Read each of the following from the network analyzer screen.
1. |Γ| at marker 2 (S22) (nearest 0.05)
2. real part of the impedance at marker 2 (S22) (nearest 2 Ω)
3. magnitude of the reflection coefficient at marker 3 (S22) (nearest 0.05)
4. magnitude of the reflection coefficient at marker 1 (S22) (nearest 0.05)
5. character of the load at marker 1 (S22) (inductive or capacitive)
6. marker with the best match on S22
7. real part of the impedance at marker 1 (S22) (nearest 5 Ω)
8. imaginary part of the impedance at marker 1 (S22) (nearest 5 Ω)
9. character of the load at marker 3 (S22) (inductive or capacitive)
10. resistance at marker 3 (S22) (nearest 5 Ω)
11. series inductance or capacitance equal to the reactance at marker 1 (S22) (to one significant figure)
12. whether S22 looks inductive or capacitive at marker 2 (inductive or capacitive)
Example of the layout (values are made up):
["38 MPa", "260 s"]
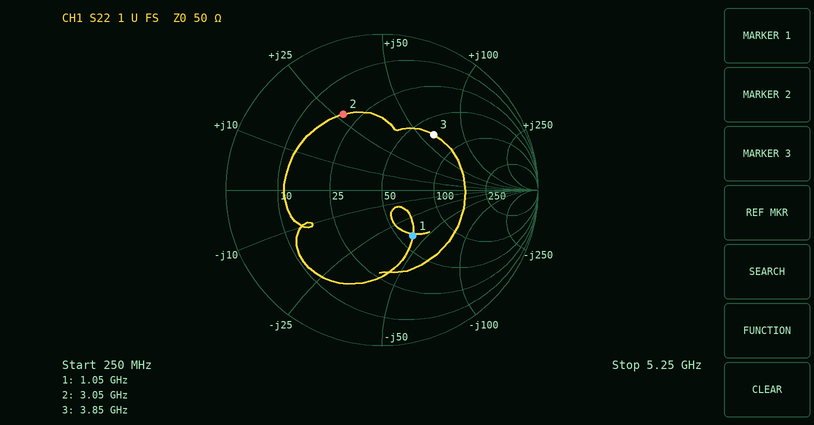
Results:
["0.55", "20 Ω", "0.50", "0.35", "capacitive", "marker 1", "60 Ω", "-40 Ω", "inductive", "65 Ω", "4 pF", "inductive"]
